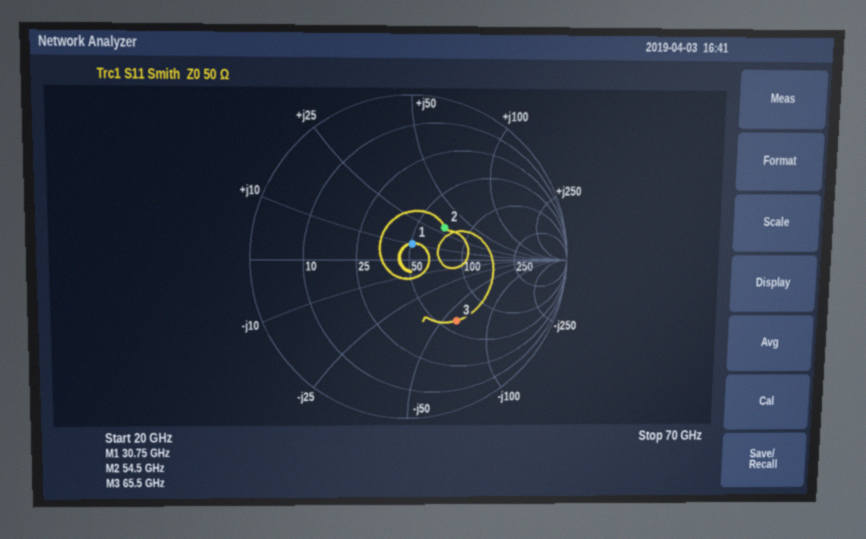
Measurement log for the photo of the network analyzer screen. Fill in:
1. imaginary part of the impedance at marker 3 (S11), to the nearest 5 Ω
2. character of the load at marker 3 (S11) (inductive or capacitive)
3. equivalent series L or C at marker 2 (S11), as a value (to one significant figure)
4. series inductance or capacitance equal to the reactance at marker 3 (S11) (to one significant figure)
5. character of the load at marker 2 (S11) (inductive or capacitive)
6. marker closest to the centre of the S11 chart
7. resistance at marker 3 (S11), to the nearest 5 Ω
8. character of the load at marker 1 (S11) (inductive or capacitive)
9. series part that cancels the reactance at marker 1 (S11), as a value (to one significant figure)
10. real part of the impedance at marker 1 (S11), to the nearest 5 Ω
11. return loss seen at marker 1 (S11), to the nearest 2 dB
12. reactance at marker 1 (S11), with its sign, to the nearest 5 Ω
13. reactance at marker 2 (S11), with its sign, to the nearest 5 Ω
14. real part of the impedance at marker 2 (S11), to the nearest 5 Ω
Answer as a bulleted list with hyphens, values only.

- -60 Ω
- capacitive
- 90 pH
- 40 fF
- inductive
- marker 1
- 60 Ω
- inductive
- 500 fF
- 50 Ω
- 20 dB
- +10 Ω
- +30 Ω
- 70 Ω
